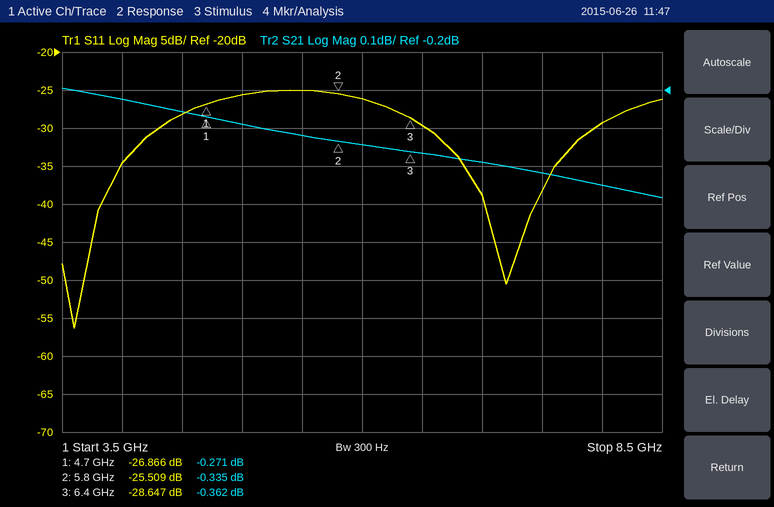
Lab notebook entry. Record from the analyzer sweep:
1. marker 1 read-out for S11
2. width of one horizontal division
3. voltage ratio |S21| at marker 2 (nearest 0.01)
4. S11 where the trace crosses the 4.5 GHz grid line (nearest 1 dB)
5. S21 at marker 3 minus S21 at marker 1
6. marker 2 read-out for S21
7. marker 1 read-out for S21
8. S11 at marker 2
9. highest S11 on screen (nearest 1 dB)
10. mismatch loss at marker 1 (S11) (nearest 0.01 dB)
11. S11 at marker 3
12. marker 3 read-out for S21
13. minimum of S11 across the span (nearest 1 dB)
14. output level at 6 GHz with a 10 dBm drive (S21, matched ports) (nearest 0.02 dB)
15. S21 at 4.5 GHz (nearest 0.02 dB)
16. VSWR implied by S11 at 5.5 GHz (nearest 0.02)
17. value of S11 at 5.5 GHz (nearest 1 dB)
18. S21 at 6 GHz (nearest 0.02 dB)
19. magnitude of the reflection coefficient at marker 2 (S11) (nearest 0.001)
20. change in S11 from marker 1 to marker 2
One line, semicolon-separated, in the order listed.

-26.866 dB; 500 MHz; 0.96; -28 dB; -0.091 dB; -0.335 dB; -0.271 dB; -25.509 dB; -25 dB; 0.01 dB; -28.647 dB; -0.362 dB; -56 dB; 9.66 dBm; -0.26 dB; 1.12; -25 dB; -0.34 dB; 0.053; 1.357 dB
